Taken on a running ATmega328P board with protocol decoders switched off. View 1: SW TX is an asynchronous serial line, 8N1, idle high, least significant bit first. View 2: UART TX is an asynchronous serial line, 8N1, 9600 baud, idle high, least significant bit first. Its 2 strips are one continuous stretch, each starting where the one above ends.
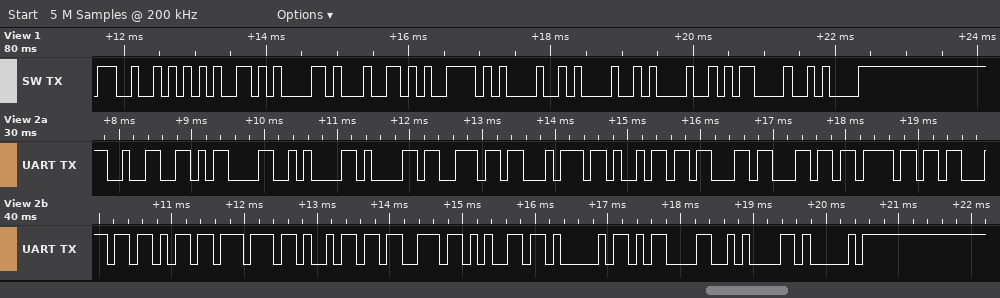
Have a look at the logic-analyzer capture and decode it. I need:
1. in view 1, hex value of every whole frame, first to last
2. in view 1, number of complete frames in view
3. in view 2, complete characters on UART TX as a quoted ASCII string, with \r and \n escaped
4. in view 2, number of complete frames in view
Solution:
0x52 0x65 0x61 0x64 0x79 0x21 0x21 0x21 0x0D 0x0A
10
"2\r\nanticlockwiseA\r\nA"
20
